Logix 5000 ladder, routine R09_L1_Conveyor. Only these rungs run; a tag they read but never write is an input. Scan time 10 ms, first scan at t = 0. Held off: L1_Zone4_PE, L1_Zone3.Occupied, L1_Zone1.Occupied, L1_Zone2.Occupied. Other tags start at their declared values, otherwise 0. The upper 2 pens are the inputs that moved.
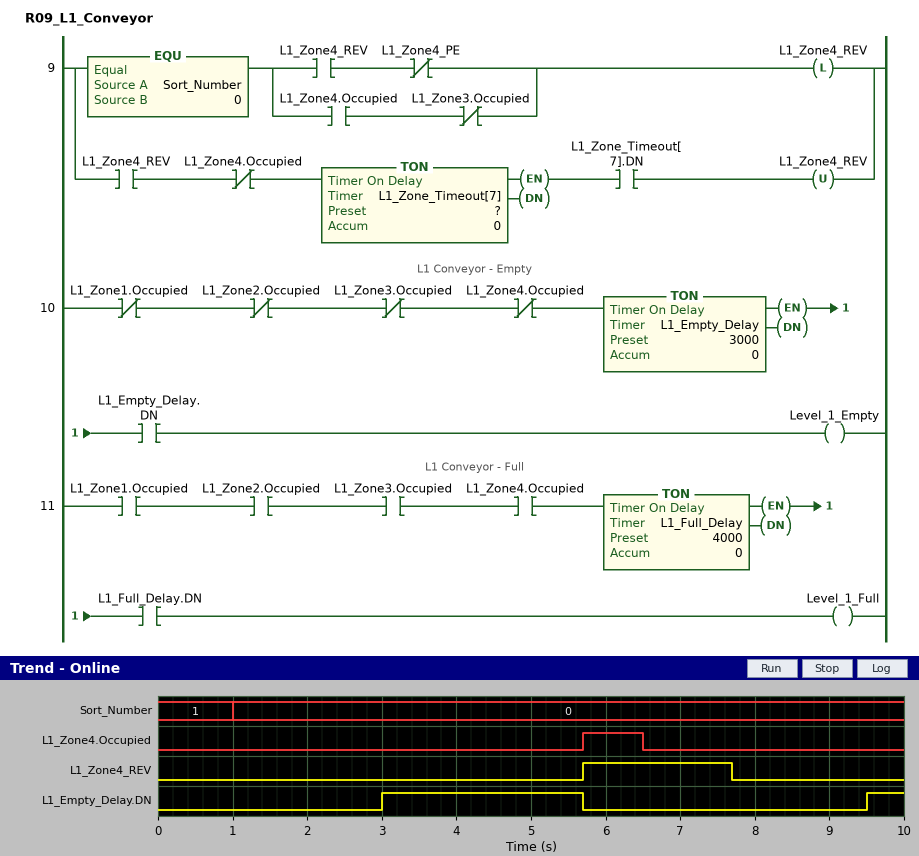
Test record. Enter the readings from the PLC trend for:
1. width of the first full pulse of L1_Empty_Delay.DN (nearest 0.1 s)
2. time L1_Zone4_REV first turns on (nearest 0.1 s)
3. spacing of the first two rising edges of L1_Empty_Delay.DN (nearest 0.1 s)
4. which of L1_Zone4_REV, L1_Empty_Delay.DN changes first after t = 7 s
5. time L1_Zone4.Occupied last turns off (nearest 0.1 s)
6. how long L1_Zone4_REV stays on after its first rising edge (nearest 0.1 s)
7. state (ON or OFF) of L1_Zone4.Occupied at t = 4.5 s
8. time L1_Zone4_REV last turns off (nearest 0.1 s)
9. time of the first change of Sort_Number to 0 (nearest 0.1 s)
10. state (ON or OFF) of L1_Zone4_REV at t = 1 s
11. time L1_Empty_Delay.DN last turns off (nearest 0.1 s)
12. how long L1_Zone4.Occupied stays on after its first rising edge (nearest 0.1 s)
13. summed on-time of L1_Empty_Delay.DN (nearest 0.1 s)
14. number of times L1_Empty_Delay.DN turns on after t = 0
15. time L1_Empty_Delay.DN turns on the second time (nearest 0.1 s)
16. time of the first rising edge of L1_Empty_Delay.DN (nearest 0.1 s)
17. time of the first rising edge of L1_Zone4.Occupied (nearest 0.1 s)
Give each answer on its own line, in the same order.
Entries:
2.7 s
5.7 s
6.5 s
L1_Zone4_REV
6.5 s
2.0 s
OFF
7.7 s
1.0 s
OFF
5.7 s
0.8 s
3.2 s
2
9.5 s
3.0 s
5.7 s
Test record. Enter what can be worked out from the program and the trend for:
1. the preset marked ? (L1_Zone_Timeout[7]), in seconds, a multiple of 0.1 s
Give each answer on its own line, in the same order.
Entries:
1.2 s
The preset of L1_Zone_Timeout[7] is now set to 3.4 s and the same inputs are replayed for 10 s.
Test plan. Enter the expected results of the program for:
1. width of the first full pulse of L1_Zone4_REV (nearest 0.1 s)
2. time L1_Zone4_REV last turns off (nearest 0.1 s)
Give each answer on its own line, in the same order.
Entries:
4.2 s
9.9 s
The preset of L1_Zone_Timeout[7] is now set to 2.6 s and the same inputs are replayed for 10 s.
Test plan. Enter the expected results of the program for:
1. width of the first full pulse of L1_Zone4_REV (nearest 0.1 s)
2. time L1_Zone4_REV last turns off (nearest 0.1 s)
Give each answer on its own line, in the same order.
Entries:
3.4 s
9.1 s
